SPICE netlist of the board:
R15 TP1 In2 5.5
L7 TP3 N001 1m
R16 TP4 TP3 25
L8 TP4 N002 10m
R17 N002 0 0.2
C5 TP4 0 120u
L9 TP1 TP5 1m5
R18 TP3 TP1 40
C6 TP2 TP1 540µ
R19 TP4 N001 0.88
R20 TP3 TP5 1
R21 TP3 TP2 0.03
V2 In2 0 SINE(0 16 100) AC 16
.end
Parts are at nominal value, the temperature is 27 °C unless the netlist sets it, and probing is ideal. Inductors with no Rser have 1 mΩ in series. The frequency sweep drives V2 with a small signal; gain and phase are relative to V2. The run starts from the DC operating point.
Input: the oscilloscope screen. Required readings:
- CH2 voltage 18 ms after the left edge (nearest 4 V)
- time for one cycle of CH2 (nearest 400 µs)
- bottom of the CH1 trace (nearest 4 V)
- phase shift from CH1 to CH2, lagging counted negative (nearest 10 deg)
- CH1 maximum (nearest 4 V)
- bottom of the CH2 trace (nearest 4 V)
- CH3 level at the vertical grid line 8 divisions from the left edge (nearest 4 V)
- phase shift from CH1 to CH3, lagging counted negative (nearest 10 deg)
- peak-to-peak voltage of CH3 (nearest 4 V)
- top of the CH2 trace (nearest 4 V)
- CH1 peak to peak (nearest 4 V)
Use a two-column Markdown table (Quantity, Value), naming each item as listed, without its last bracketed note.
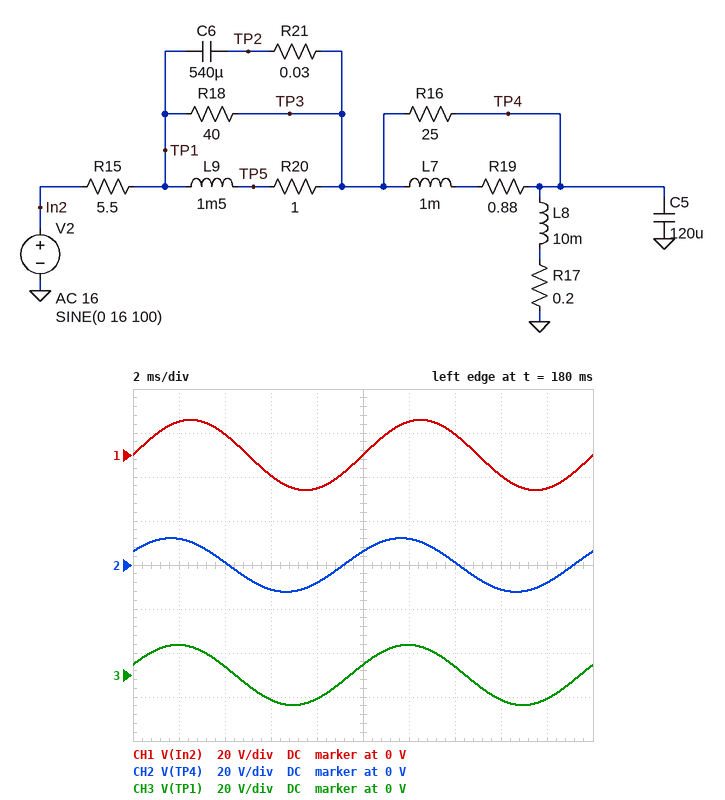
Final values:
| Quantity | Value |
|---|---|
| CH2 voltage 18 ms after the left edge | -8 V |
| time for one cycle of CH2 | 10.0 ms |
| bottom of the CH1 trace | -16 V |
| phase shift from CH1 to CH2, lagging counted negative | 30 deg |
| CH1 maximum | 16 V |
| bottom of the CH2 trace | -12 V |
| CH3 level at the vertical grid line 8 divisions from the left edge | -12 V |
| phase shift from CH1 to CH3, lagging counted negative | 20 deg |
| peak-to-peak voltage of CH3 | 28 V |
| top of the CH2 trace | 12 V |
| CH1 peak to peak | 32 V |
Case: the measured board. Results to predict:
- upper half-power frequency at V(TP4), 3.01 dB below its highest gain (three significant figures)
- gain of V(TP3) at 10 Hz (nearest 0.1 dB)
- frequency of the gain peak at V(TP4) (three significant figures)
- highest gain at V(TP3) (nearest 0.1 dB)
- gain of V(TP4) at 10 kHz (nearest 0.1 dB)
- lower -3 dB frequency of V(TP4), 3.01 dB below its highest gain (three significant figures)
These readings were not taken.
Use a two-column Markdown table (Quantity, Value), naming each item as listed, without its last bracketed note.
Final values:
| Quantity | Value |
|---|---|
| upper half-power frequency at V(TP4), 3.01 dB below its highest gain | 277 Hz |
| gain of V(TP3) at 10 Hz | -15.6 dB |
| frequency of the gain peak at V(TP4) | 150 Hz |
| highest gain at V(TP3) | -0.2 dB |
| gain of V(TP4) at 10 kHz | -46.6 dB |
| lower -3 dB frequency of V(TP4), 3.01 dB below its highest gain | 89.6 Hz |
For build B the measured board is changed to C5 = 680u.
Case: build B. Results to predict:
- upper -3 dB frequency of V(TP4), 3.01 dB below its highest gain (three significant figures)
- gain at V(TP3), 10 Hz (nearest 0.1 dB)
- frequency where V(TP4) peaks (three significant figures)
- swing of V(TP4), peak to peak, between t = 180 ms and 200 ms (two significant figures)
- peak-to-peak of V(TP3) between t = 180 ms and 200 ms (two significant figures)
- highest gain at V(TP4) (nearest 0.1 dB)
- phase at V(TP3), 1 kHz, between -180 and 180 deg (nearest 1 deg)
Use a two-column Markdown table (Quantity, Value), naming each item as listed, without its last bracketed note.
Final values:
| Quantity | Value |
|---|---|
| upper -3 dB frequency of V(TP4), 3.01 dB below its highest gain | 82.5 Hz |
| gain at V(TP3), 10 Hz | -15.5 dB |
| frequency where V(TP4) peaks | 63.3 Hz |
| swing of V(TP4), peak to peak, between t = 180 ms and 200 ms | 14 V |
| peak-to-peak of V(TP3) between t = 180 ms and 200 ms | 12 V |
| highest gain at V(TP4) | -0.8 dB |
| phase at V(TP3), 1 kHz, between -180 and 180 deg | 35 deg |
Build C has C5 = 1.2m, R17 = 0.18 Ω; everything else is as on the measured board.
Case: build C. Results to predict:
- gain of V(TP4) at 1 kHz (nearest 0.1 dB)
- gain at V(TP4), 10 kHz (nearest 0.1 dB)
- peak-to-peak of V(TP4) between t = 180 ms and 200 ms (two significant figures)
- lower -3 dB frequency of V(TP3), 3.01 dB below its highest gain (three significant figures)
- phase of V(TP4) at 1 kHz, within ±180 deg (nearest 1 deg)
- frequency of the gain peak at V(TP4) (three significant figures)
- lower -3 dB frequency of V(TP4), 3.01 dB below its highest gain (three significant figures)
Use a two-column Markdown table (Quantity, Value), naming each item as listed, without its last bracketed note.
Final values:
| Quantity | Value |
|---|---|
| gain of V(TP4) at 1 kHz | -36.9 dB |
| gain at V(TP4), 10 kHz | -66.6 dB |
| peak-to-peak of V(TP4) between t = 180 ms and 200 ms | 6.7 V |
| lower -3 dB frequency of V(TP3), 3.01 dB below its highest gain | 36.8 Hz |
| phase of V(TP4) at 1 kHz, within ±180 deg | -123 deg |
| frequency of the gain peak at V(TP4) | 47.1 Hz |
| lower -3 dB frequency of V(TP4), 3.01 dB below its highest gain | 37.7 Hz |
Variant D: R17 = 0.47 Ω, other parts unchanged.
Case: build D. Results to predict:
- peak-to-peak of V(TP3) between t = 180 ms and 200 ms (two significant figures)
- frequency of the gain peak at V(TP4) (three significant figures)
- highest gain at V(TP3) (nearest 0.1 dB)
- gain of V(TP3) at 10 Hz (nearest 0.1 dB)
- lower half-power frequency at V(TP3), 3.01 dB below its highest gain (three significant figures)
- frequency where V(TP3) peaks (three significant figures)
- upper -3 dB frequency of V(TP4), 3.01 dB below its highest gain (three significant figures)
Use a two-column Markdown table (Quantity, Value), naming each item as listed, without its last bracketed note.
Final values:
| Quantity | Value |
|---|---|
| peak-to-peak of V(TP3) between t = 180 ms and 200 ms | 25 V |
| frequency of the gain peak at V(TP4) | 151 Hz |
| highest gain at V(TP3) | -0.4 dB |
| gain of V(TP3) at 10 Hz | -14.4 dB |
| lower half-power frequency at V(TP3), 3.01 dB below its highest gain | 82.2 Hz |
| frequency where V(TP3) peaks | 146 Hz |
| upper -3 dB frequency of V(TP4), 3.01 dB below its highest gain | 290 Hz |
